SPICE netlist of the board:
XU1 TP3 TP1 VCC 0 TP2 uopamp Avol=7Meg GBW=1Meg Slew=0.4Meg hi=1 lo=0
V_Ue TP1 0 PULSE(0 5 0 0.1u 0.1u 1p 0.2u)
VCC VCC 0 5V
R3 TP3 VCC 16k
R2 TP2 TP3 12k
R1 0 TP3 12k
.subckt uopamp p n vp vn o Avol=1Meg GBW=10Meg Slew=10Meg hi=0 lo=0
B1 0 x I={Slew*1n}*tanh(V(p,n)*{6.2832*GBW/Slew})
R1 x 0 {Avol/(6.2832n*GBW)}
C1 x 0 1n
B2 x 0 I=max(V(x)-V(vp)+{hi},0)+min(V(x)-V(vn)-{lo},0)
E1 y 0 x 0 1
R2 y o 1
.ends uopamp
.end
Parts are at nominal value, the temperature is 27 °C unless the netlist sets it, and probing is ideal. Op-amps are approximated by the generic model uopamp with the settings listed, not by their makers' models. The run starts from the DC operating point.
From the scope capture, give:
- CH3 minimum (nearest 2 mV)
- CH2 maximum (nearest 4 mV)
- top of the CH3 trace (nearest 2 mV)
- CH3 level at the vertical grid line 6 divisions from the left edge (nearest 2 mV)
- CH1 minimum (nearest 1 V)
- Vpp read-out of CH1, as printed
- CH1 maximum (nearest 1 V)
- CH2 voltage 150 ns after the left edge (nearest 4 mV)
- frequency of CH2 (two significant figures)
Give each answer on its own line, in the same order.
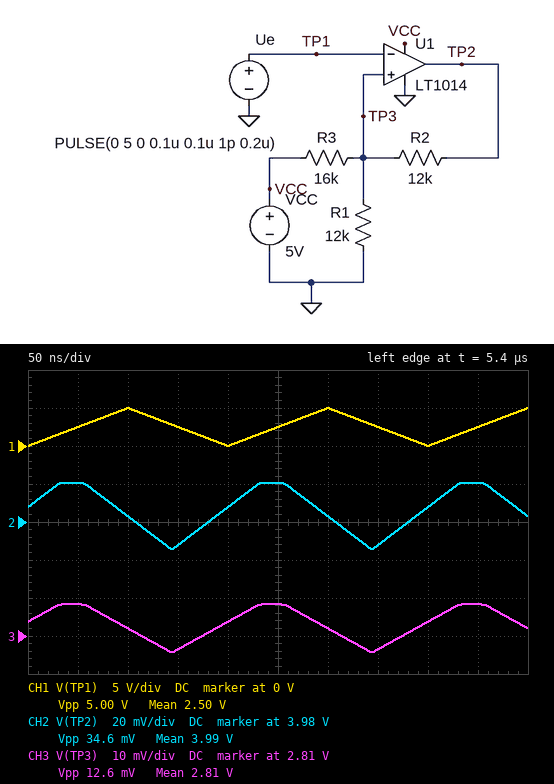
2.806 V
4.000 V
2.818 V
2.812 V
0 V
5.00 V
5 V
3.968 V
5.0 MHz
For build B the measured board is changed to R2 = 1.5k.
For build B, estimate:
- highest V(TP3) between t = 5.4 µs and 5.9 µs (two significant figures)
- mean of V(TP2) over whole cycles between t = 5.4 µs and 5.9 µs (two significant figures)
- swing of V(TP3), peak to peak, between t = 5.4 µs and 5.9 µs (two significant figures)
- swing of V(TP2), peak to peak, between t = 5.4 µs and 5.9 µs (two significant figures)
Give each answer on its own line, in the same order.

3.7 V
4.0 V
17 mV
21 mV
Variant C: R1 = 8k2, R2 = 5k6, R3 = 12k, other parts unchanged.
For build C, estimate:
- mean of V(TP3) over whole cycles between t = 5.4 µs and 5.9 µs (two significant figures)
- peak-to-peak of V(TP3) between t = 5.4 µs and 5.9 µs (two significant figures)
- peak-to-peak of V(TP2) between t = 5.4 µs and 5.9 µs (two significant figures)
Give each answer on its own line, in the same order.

2.9 V
15 mV
33 mV
